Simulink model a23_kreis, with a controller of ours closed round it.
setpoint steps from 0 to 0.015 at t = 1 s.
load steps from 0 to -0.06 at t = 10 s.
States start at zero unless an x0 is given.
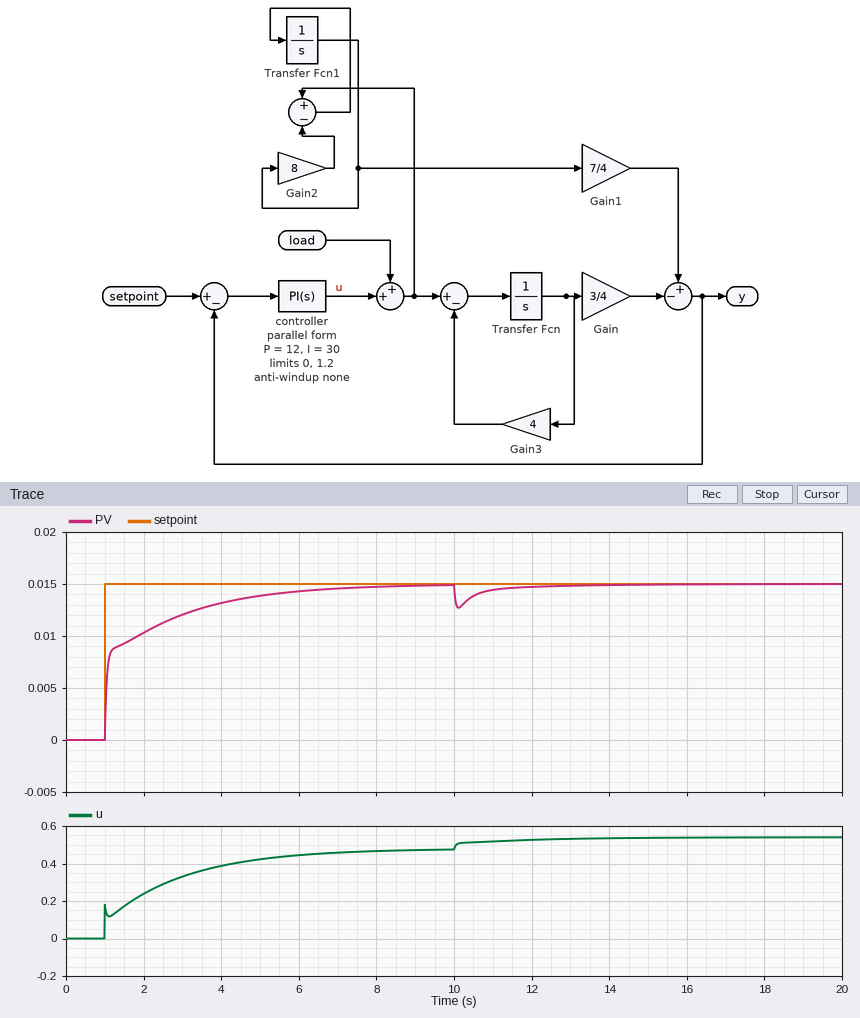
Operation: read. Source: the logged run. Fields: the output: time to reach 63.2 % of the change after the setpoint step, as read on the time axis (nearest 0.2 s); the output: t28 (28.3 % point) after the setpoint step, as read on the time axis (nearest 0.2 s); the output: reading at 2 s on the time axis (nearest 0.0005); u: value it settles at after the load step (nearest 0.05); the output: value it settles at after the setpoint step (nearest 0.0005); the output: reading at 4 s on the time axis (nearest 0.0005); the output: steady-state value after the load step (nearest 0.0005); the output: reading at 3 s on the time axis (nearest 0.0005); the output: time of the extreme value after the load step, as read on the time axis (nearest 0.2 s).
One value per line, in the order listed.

1.6 s
1.0 s
0.0105
0.55
0.0150
0.0130
0.0150
0.0120
10.2 s
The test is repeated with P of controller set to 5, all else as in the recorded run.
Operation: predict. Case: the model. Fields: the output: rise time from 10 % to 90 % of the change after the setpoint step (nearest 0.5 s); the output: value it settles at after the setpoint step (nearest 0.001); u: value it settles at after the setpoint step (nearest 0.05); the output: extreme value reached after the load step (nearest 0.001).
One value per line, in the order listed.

3.0 s
0.015
0.50
0.012
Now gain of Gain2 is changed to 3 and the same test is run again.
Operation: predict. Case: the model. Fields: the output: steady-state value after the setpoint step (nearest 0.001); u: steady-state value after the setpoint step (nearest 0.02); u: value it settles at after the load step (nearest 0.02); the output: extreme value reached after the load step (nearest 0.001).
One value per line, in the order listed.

0.015
0.04
0.10
0.012
